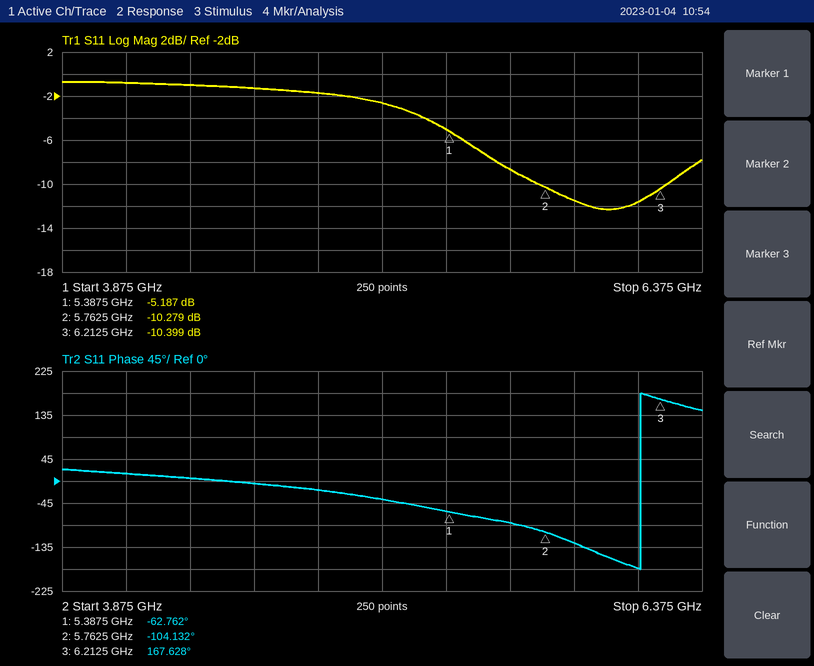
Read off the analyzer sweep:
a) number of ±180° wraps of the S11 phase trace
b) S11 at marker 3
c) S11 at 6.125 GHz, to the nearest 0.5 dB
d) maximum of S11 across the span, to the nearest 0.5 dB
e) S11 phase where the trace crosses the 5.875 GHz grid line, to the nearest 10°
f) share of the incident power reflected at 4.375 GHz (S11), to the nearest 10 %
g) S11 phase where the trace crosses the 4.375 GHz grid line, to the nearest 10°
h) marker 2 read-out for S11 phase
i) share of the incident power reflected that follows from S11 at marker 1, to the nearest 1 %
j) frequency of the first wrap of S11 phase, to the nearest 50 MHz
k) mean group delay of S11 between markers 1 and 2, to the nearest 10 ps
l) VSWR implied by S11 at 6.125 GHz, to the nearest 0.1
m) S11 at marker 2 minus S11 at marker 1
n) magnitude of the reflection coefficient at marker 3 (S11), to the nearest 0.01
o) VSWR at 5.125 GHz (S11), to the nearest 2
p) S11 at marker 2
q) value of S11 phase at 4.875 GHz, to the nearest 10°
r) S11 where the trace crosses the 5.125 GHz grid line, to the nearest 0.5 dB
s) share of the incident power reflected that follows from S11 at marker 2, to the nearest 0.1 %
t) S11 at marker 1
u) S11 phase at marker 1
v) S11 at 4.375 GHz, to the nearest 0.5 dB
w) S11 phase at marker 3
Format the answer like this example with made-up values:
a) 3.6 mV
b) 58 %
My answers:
a) 1
b) -10.399 dB
c) -11.5 dB
d) -0.5 dB
e) -130°
f) 80 %
g) 10°
h) -104.132°
i) 30 %
j) 6.15 GHz
k) 310 ps
l) 1.7
m) -5.092 dB
n) 0.30
o) 6
p) -10.279 dB
q) -20°
r) -2.5 dB
s) 9.4 %
t) -5.187 dB
u) -62.762°
v) -1.0 dB
w) 167.628°
